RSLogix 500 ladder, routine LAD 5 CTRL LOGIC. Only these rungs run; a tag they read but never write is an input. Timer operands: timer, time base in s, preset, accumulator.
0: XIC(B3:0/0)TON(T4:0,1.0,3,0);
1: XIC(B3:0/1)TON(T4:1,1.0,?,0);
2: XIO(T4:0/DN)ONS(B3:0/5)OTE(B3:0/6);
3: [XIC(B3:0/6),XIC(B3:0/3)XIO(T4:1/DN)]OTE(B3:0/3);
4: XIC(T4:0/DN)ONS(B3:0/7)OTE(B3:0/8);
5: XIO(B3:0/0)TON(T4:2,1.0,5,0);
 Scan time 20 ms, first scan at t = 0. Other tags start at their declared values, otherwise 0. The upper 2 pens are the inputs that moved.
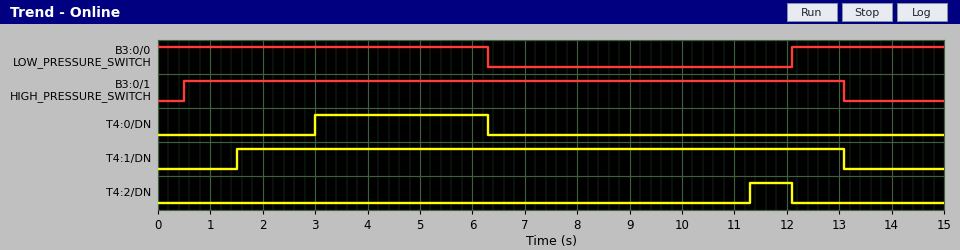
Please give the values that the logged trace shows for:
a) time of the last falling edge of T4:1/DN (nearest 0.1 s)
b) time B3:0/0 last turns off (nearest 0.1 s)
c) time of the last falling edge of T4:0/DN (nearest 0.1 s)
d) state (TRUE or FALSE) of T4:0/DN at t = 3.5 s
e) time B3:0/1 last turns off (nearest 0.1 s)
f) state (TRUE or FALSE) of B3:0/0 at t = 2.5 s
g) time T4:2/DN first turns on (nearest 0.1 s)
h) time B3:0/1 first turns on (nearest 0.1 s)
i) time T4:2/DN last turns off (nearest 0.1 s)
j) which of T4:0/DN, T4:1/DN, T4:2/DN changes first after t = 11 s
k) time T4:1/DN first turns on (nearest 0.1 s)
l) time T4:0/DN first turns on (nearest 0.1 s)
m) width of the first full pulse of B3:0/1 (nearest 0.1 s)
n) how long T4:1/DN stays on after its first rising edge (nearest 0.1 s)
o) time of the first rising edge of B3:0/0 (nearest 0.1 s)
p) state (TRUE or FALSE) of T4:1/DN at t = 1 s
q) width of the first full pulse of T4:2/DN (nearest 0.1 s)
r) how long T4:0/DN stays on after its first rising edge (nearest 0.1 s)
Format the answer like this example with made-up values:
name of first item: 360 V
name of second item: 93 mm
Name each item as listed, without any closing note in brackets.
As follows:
time of the last falling edge of T4:1/DN: 13.1 s
time B3:0/0 last turns off: 6.3 s
time of the last falling edge of T4:0/DN: 6.3 s
state (TRUE or FALSE) of T4:0/DN at t = 3.5 s: TRUE
time B3:0/1 last turns off: 13.1 s
state (TRUE or FALSE) of B3:0/0 at t = 2.5 s: TRUE
time T4:2/DN first turns on: 11.3 s
time B3:0/1 first turns on: 0.5 s
time T4:2/DN last turns off: 12.1 s
which of T4:0/DN, T4:1/DN, T4:2/DN changes first after t = 11 s: T4:2/DN
time T4:1/DN first turns on: 1.5 s
time T4:0/DN first turns on: 3.0 s
width of the first full pulse of B3:0/1: 12.6 s
how long T4:1/DN stays on after its first rising edge: 11.6 s
time of the first rising edge of B3:0/0: 12.1 s
state (TRUE or FALSE) of T4:1/DN at t = 1 s: FALSE
width of the first full pulse of T4:2/DN: 0.8 s
how long T4:0/DN stays on after its first rising edge: 3.3 s
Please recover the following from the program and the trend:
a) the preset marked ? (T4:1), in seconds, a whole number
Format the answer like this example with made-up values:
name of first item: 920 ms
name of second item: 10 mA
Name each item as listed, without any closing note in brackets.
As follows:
the preset marked ? (T4:1), in seconds, a whole number: 1 s
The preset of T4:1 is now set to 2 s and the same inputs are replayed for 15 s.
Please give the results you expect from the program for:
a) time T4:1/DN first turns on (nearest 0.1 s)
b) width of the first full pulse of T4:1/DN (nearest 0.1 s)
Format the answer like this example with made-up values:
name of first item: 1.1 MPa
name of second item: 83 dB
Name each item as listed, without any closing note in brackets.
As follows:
time T4:1/DN first turns on: 2.5 s
width of the first full pulse of T4:1/DN: 10.6 s
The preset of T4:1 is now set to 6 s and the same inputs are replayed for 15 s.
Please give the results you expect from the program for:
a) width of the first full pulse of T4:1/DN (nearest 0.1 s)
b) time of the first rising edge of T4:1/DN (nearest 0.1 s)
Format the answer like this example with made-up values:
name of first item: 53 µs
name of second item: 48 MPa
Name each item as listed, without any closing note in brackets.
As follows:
width of the first full pulse of T4:1/DN: 6.6 s
time of the first rising edge of T4:1/DN: 6.5 s
